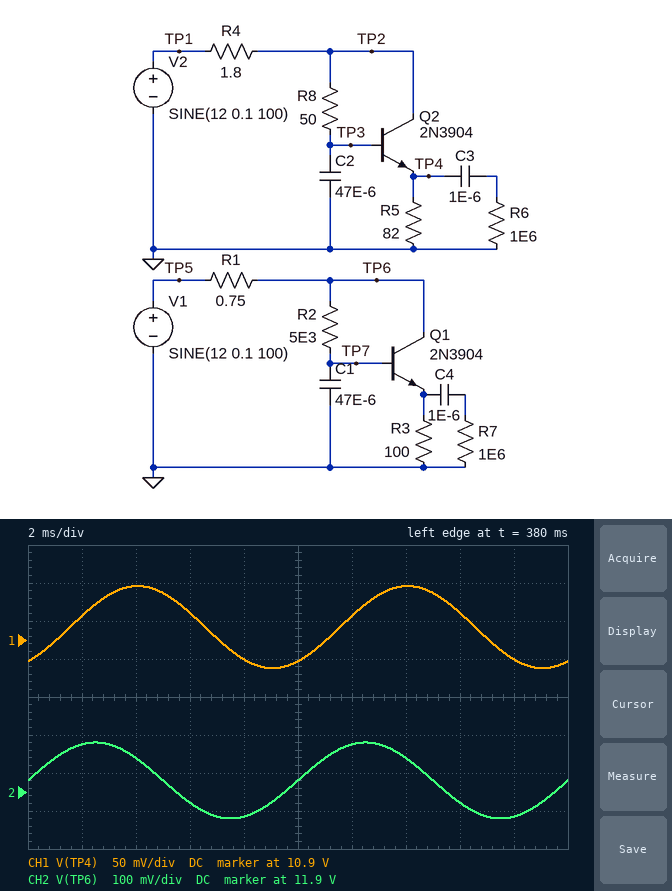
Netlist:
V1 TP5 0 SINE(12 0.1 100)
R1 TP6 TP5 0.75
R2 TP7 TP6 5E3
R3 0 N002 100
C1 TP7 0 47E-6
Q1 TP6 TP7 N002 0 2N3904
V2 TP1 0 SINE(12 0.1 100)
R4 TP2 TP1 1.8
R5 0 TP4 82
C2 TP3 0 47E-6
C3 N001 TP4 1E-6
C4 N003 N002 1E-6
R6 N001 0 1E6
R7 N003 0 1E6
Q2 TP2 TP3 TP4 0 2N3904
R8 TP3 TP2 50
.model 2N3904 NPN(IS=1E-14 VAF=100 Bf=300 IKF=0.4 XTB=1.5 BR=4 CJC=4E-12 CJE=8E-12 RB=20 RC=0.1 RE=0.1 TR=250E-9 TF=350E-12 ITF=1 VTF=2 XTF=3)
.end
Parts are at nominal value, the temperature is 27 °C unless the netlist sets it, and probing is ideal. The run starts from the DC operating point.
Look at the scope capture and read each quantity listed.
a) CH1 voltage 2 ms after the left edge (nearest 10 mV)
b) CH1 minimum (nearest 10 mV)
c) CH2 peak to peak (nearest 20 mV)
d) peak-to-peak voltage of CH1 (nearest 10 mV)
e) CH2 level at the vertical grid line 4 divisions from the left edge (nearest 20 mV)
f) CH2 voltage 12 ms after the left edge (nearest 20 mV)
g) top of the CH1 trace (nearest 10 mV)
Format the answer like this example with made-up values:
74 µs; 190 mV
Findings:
10.93 V; 10.86 V; 200 mV; 110 mV; 11.84 V; 12.02 V; 10.97 V
